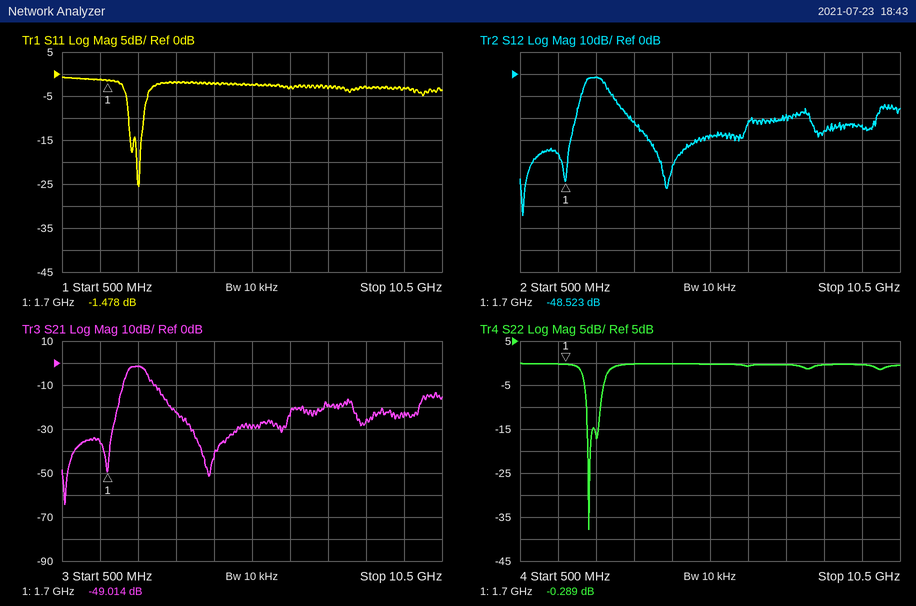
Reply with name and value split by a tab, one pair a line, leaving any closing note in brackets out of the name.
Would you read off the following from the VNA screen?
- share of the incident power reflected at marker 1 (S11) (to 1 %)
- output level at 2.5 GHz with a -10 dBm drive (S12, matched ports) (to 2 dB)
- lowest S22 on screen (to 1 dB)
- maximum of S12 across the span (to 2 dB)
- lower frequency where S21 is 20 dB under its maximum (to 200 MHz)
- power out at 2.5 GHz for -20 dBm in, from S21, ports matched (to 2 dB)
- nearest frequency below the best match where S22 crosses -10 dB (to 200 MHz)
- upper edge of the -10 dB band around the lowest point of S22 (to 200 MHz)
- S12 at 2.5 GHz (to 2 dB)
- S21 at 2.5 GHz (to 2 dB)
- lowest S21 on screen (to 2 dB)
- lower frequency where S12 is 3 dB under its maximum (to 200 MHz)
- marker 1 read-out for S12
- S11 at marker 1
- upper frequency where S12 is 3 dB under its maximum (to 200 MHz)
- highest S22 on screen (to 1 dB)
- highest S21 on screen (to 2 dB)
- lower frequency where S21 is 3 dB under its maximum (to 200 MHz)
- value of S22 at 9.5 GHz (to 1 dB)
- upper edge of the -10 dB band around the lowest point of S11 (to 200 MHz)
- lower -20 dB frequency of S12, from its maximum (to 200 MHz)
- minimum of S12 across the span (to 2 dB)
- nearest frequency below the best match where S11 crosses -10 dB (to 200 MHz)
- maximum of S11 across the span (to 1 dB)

share of the incident power reflected at marker 1 (S11)	71 %
output level at 2.5 GHz with a -10 dBm drive (S12, matched ports)	-12 dBm
lowest S22 on screen	-38 dB
maximum of S12 across the span	-2 dB
lower frequency where S21 is 20 dB under its maximum	2.0 GHz
power out at 2.5 GHz for -20 dBm in, from S21, ports matched	-22 dBm
nearest frequency below the best match where S22 crosses -10 dB	2.2 GHz
upper edge of the -10 dB band around the lowest point of S22	2.6 GHz
S12 at 2.5 GHz	-2 dB
S21 at 2.5 GHz	-2 dB
lowest S21 on screen	-64 dB
lower frequency where S12 is 3 dB under its maximum	2.2 GHz
marker 1 read-out for S12	-48.523 dB
S11 at marker 1	-1.478 dB
upper frequency where S12 is 3 dB under its maximum	2.8 GHz
highest S22 on screen	0 dB
highest S21 on screen	-2 dB
lower frequency where S21 is 3 dB under its maximum	2.2 GHz
value of S22 at 9.5 GHz	0 dB
upper edge of the -10 dB band around the lowest point of S11	2.6 GHz
lower -20 dB frequency of S12, from its maximum	2.0 GHz
minimum of S12 across the span	-64 dB
nearest frequency below the best match where S11 crosses -10 dB	2.2 GHz
maximum of S11 across the span	-1 dB
